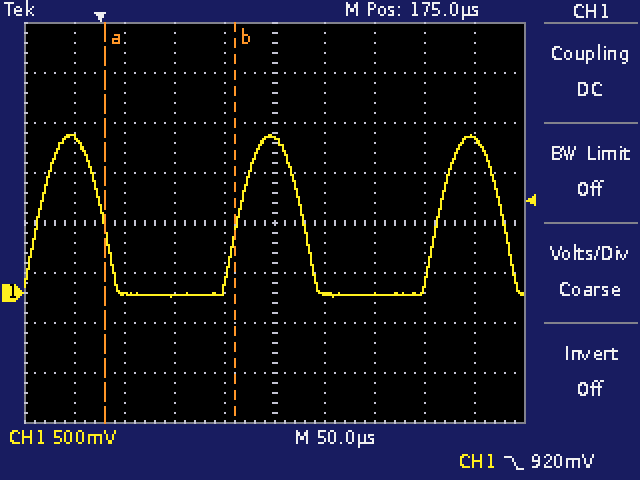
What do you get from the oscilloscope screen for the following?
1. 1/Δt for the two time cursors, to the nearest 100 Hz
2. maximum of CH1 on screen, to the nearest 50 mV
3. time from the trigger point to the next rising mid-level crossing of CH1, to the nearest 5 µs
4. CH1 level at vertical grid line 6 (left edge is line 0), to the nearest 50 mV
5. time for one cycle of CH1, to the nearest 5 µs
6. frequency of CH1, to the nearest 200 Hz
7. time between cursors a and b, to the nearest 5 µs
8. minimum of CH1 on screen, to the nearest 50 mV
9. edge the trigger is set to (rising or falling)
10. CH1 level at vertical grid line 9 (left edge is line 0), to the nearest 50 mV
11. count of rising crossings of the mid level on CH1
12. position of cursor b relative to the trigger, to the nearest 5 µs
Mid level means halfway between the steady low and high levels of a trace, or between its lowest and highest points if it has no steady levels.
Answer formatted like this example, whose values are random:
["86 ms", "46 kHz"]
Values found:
["7.7 kHz", "1.60 V", "140 µs", "0 mV", "200 µs", "5.0 kHz", "130 µs", "-50 mV", "falling", "1.55 V", "3", "+135 µs"]
